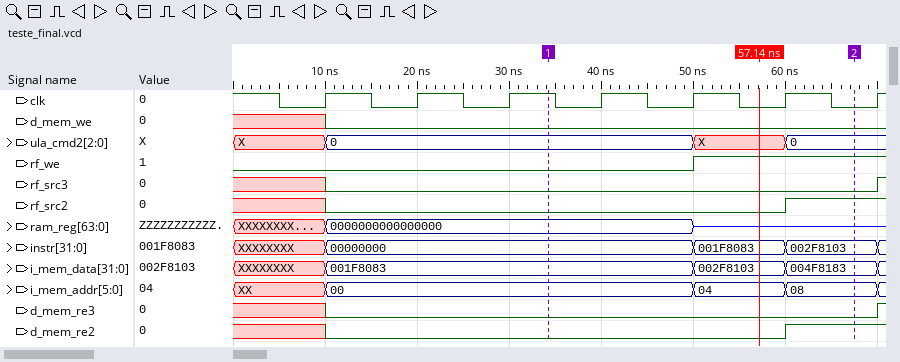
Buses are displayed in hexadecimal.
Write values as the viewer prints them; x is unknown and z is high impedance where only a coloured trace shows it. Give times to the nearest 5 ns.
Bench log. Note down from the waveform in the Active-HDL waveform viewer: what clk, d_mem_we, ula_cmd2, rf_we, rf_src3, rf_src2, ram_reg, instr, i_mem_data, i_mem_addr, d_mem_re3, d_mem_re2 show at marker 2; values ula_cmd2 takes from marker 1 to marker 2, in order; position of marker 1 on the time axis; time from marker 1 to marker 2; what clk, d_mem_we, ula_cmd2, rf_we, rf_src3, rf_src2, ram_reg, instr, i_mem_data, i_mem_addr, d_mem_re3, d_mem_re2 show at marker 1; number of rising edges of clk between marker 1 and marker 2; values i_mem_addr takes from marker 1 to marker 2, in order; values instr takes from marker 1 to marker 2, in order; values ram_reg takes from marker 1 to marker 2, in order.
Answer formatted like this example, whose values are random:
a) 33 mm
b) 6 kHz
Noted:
a) clk=0, d_mem_we=0, ula_cmd2=0, rf_we=1, rf_src3=0, rf_src2=1, ram_reg=z, instr=002F8103, i_mem_data=004F8183, i_mem_addr=08, d_mem_re3=0, d_mem_re2=1
b) 0, X, 0
c) 35 ns
d) 35 ns
e) clk=1, d_mem_we=0, ula_cmd2=0, rf_we=0, rf_src3=0, rf_src2=0, ram_reg=0000000000000000, instr=00000000, i_mem_data=001F8083, i_mem_addr=00, d_mem_re3=0, d_mem_re2=0
f) 3
g) 00, 04, 08
h) 00000000, 001F8083, 002F8103
i) 0000000000000000, z
